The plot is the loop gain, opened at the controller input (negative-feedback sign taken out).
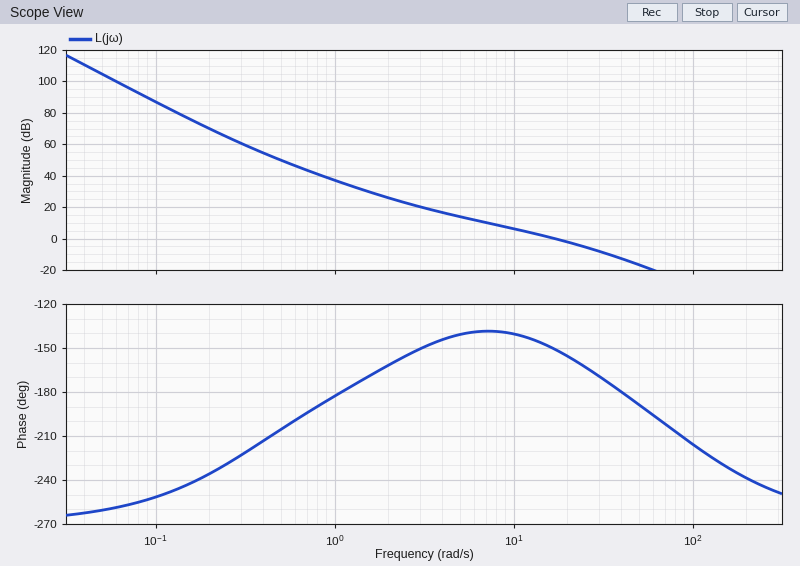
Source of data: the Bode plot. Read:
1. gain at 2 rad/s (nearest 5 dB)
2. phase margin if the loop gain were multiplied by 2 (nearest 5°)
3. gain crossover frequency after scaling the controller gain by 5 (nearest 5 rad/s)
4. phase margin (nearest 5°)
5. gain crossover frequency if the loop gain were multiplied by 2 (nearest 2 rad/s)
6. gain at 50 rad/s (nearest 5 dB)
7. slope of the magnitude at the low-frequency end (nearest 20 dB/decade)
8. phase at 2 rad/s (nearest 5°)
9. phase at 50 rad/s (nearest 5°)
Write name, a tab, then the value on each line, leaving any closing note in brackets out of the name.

gain at 2 rad/s	25 dB
phase margin if the loop gain were multiplied by 2	15°
gain crossover frequency after scaling the controller gain by 5	45 rad/s
phase margin	30°
gain crossover frequency if the loop gain were multiplied by 2	26 rad/s
gain at 50 rad/s	-15 dB
slope of the magnitude at the low-frequency end	-60 dB/decade
phase at 2 rad/s	-160°
phase at 50 rad/s	-190°
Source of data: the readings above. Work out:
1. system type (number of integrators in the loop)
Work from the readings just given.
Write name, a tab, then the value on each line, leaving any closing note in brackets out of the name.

system type	3
